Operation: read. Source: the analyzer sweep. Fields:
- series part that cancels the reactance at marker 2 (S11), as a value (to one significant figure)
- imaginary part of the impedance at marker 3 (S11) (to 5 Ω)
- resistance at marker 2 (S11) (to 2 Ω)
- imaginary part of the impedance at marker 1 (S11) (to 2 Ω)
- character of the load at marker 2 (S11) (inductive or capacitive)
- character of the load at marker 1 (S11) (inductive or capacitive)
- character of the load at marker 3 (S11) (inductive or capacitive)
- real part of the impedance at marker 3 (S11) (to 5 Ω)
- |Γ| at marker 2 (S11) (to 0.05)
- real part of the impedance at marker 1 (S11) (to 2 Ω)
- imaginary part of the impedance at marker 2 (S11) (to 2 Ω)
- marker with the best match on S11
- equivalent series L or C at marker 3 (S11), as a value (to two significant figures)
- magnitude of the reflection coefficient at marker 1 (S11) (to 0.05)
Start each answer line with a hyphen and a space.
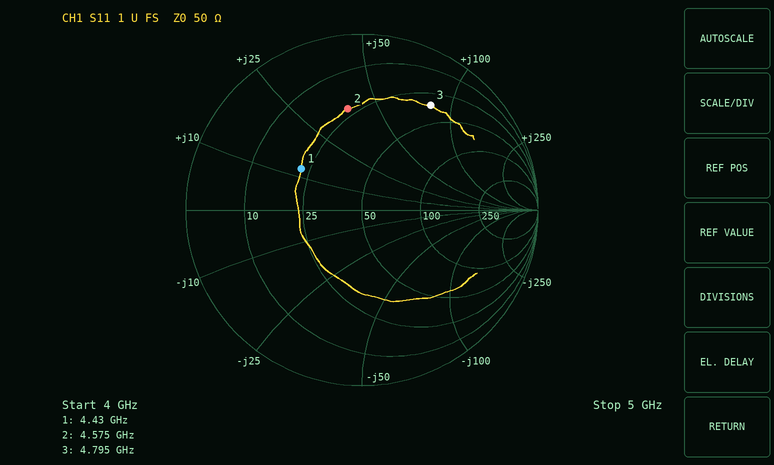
- 900 fF
- +80 Ω
- 22 Ω
- +12 Ω
- inductive
- inductive
- inductive
- 35 Ω
- 0.60
- 22 Ω
- +38 Ω
- marker 1
- 2.7 nH
- 0.40
